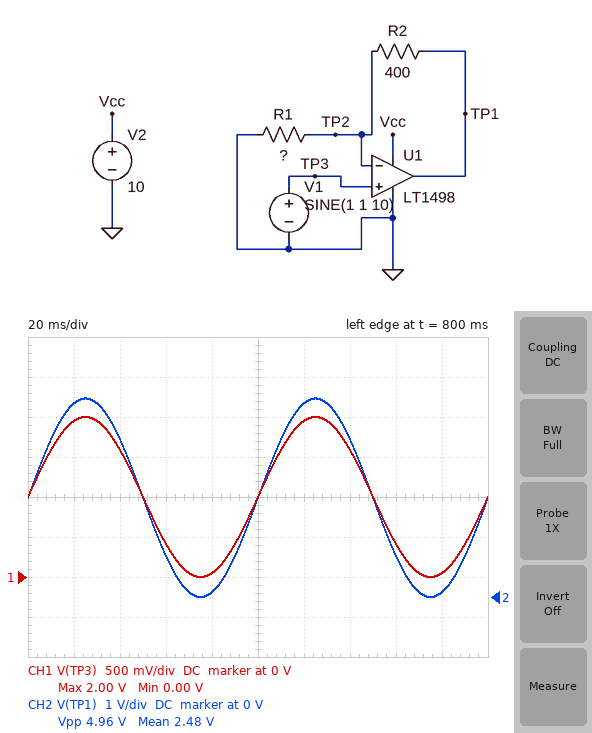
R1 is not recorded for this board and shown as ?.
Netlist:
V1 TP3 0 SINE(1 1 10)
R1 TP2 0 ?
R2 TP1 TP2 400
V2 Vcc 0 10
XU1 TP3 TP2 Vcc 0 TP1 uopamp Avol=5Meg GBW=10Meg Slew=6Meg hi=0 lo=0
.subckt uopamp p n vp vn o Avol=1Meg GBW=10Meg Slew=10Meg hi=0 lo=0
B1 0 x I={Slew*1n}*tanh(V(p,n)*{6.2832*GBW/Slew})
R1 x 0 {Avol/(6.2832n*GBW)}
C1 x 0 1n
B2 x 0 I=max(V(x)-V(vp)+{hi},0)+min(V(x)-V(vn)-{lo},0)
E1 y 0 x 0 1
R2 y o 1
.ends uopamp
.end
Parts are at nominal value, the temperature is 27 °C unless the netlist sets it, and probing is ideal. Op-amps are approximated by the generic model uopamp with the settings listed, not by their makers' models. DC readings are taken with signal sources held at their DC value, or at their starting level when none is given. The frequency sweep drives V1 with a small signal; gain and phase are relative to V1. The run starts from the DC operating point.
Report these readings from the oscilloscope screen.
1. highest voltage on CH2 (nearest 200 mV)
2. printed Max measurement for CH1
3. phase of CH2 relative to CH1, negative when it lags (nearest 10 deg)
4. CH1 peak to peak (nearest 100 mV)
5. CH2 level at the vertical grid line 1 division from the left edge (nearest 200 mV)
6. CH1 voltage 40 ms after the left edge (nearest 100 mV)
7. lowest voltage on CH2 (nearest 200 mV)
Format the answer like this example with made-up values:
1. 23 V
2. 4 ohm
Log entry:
1. 5.0 V
2. 2.00 V
3. 0 deg
4. 2.0 V
5. 4.8 V
6. 1.6 V
7. 0 V
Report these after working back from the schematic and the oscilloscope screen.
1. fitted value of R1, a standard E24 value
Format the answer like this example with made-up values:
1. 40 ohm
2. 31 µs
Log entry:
1. 270 Ω
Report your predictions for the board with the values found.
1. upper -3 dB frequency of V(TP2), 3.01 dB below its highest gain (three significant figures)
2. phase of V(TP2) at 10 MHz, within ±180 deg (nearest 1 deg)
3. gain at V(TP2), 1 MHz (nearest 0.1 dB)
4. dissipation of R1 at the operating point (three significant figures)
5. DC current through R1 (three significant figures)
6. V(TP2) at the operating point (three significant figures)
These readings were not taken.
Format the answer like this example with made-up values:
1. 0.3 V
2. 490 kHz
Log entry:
1. 4.02 MHz
2. -68 deg
3. -0.3 dB
4. 3.70 mW
5. 3.70 mA
6. 1.00 V
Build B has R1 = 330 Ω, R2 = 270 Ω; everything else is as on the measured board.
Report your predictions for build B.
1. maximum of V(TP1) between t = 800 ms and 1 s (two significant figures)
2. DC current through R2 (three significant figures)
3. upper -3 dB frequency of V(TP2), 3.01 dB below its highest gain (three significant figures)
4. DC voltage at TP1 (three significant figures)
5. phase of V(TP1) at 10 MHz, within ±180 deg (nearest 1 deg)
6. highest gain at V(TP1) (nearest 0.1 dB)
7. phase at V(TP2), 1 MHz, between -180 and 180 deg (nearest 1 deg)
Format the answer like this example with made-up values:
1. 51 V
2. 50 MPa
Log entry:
1. 3.6 V
2. 3.03 mA
3. 5.49 MHz
4. 1.82 V
5. -61 deg
6. 5.2 dB
7. -10 deg
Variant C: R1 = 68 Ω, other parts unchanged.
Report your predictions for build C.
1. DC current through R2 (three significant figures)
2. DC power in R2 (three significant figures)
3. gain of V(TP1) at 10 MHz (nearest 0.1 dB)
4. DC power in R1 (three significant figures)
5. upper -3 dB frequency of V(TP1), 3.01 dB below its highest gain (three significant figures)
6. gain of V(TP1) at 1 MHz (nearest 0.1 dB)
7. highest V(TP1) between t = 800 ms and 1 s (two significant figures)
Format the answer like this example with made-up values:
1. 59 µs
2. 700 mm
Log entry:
1. 14.7 mA
2. 86.5 mW
3. -0.1 dB
4. 14.7 mW
5. 1.45 MHz
6. 15.1 dB
7. 10 V
